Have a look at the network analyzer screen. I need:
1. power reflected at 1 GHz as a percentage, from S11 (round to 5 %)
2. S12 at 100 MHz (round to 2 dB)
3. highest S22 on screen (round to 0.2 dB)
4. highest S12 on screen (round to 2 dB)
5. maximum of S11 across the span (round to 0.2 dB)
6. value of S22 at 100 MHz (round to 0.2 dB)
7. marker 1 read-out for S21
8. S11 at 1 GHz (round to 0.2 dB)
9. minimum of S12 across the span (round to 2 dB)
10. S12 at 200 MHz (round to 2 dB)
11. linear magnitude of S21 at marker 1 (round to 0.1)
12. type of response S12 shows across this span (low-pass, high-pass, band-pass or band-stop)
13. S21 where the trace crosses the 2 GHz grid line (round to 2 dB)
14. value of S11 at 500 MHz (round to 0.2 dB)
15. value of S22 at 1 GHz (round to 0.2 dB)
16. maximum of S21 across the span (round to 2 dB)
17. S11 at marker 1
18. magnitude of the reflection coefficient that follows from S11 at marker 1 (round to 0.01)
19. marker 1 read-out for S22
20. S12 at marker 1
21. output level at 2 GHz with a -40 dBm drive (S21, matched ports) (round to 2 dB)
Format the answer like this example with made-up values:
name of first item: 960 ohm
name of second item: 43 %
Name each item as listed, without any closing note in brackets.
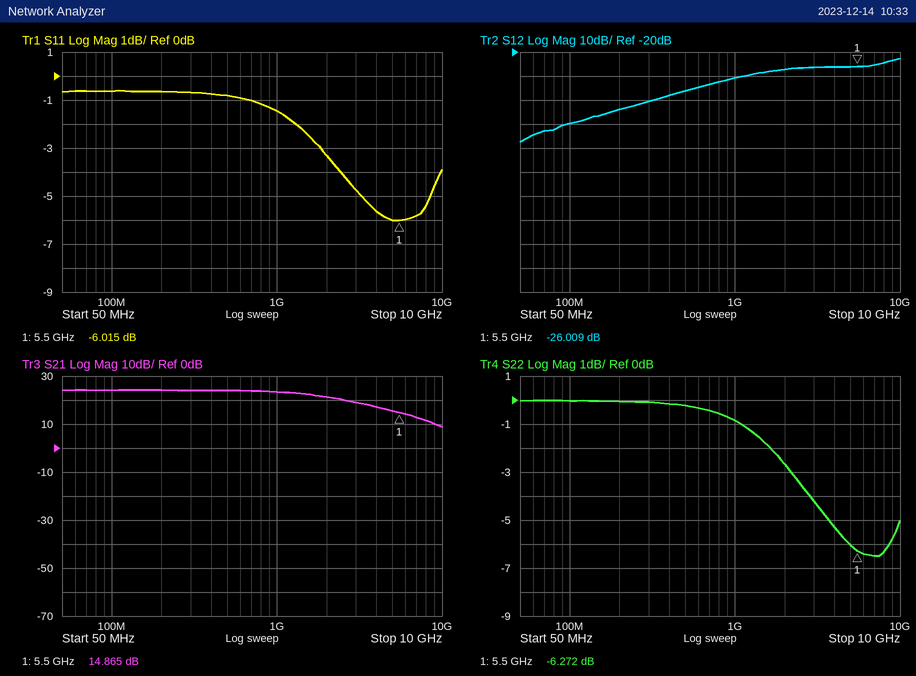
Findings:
power reflected at 1 GHz as a percentage, from S11: 70 %
S12 at 100 MHz: -50 dB
highest S22 on screen: 0.0 dB
highest S12 on screen: -22 dB
maximum of S11 across the span: -0.6 dB
value of S22 at 100 MHz: 0.0 dB
marker 1 read-out for S21: 14.865 dB
S11 at 1 GHz: -1.4 dB
minimum of S12 across the span: -58 dB
S12 at 200 MHz: -44 dB
linear magnitude of S21 at marker 1: 5.5
type of response S12 shows across this span: high-pass
S21 where the trace crosses the 2 GHz grid line: 22 dB
value of S11 at 500 MHz: -0.8 dB
value of S22 at 1 GHz: -0.8 dB
maximum of S21 across the span: 24 dB
S11 at marker 1: -6.015 dB
magnitude of the reflection coefficient that follows from S11 at marker 1: 0.50
marker 1 read-out for S22: -6.272 dB
S12 at marker 1: -26.009 dB
output level at 2 GHz with a -40 dBm drive (S21, matched ports): -18 dBm
